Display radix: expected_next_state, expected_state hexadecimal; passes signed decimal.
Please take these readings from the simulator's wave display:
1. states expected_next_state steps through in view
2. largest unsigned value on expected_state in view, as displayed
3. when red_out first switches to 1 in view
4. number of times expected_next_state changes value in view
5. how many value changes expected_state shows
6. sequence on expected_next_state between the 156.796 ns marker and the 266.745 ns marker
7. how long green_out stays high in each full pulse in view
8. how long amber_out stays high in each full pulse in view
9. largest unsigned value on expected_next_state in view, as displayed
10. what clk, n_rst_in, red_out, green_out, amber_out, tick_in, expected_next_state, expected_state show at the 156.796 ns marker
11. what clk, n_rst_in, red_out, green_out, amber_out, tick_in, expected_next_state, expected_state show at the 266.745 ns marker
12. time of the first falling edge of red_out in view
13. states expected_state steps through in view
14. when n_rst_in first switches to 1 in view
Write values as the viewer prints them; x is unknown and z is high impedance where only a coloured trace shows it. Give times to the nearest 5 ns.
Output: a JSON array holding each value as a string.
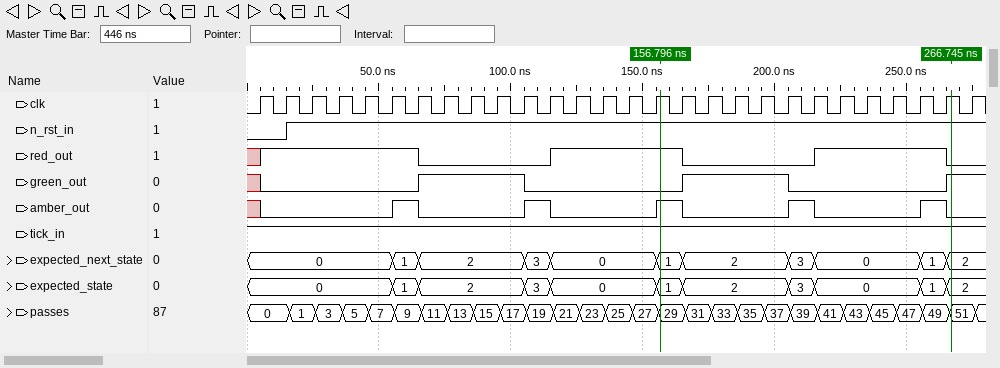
["0, 1, 2, 3, 0, 1, 2, 3, 0, 1, 2", "3", "5 ns", "10", "10", "1, 2, 3, 0, 1, 2", "40 ns, 40 ns", "10 ns, 10 ns, 10 ns, 10 ns, 10 ns", "3", "clk=1, n_rst_in=1, red_out=1, green_out=0, amber_out=1, tick_in=1, expected_next_state=1, expected_state=1", "clk=1, n_rst_in=1, red_out=0, green_out=1, amber_out=0, tick_in=1, expected_next_state=2, expected_state=2", "65 ns", "0, 1, 2, 3, 0, 1, 2, 3, 0, 1, 2", "15 ns"]
